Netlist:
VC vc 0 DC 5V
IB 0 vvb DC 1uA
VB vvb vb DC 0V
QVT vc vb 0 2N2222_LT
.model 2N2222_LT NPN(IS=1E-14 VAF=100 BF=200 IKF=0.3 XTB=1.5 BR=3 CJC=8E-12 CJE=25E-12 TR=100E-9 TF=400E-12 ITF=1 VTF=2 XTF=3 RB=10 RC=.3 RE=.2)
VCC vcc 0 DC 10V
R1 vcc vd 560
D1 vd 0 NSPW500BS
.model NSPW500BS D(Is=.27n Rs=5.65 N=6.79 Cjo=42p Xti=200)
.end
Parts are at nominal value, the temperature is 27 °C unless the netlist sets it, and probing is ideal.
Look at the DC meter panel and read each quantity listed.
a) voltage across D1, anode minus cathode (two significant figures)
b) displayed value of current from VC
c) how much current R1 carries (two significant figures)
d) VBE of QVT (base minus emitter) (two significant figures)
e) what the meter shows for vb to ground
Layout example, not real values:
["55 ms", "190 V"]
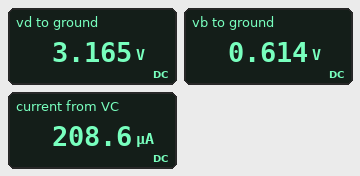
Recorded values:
["3.2 V", "208.6 µA", "12 mA", "610 mV", "0.614 V"]
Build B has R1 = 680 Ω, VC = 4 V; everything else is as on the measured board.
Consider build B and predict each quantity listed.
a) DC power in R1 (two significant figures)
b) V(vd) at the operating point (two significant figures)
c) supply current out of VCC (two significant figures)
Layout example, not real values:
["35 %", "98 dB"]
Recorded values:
["70 mW", "3.1 V", "10 mA"]
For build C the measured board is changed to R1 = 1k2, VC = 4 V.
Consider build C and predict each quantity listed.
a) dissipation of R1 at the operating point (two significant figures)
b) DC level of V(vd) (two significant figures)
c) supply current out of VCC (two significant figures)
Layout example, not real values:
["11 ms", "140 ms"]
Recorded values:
["41 mW", "3.0 V", "5.8 mA"]
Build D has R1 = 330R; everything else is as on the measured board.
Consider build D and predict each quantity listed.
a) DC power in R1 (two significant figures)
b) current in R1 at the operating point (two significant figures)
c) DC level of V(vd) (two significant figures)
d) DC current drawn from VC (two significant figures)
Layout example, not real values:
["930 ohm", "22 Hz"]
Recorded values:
["140 mW", "20 mA", "3.3 V", "210 µA"]
